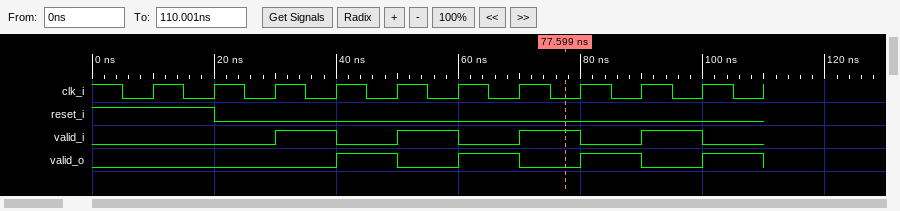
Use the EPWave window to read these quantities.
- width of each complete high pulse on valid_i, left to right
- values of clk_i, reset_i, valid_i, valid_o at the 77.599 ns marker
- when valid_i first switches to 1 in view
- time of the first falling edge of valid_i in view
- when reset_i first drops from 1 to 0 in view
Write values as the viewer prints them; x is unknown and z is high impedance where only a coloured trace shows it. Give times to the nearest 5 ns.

10 ns, 10 ns, 10 ns, 10 ns
clk_i=0, reset_i=0, valid_i=1, valid_o=0
30 ns
40 ns
20 ns
